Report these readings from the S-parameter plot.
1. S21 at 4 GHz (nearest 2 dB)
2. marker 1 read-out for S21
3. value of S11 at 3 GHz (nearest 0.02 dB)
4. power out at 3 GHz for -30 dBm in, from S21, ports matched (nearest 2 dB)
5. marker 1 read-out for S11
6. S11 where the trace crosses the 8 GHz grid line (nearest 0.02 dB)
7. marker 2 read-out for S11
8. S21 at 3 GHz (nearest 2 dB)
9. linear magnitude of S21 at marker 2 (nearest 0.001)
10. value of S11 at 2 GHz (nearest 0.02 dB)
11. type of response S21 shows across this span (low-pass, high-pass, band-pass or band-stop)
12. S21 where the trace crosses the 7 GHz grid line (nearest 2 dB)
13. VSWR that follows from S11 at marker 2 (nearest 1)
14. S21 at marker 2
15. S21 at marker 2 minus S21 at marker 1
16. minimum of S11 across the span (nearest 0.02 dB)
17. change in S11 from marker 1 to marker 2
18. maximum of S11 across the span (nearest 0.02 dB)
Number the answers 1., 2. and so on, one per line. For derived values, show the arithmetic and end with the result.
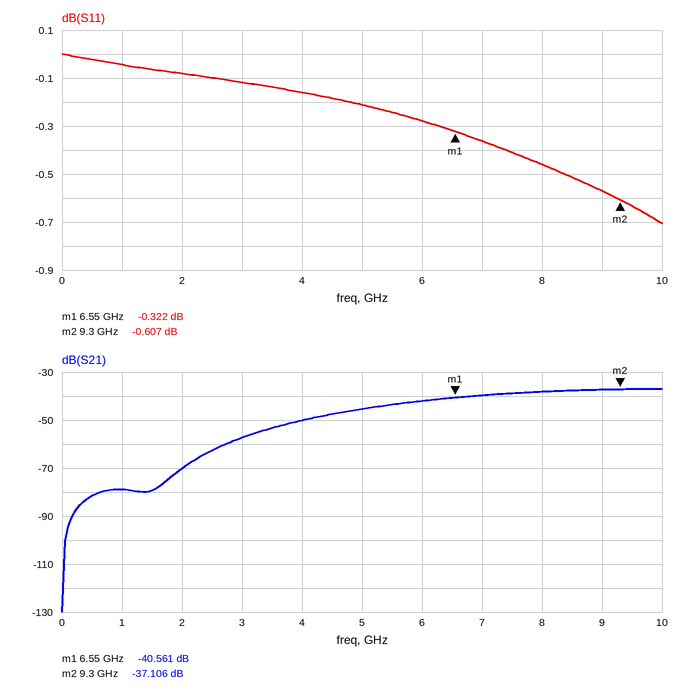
1. -50 dB
2. -40.561 dB
3. -0.12 dB
4. -30 dBm + (-58 dB) = -88 dBm
5. -0.322 dB
6. -0.46 dB
7. -0.607 dB
8. -58 dB
9. 10^(-37.106/20) ≈ 0.014
10. -0.08 dB
11. high-pass
12. -40 dB
13. (1 + 0.9325)/(1 − 0.9325) ≈ 29
14. -37.106 dB
15. -37.106 − (-40.561) = 3.455 dB
16. -0.70 dB
17. -0.607 − (-0.322) = -0.285 dB
18. 0.00 dB
